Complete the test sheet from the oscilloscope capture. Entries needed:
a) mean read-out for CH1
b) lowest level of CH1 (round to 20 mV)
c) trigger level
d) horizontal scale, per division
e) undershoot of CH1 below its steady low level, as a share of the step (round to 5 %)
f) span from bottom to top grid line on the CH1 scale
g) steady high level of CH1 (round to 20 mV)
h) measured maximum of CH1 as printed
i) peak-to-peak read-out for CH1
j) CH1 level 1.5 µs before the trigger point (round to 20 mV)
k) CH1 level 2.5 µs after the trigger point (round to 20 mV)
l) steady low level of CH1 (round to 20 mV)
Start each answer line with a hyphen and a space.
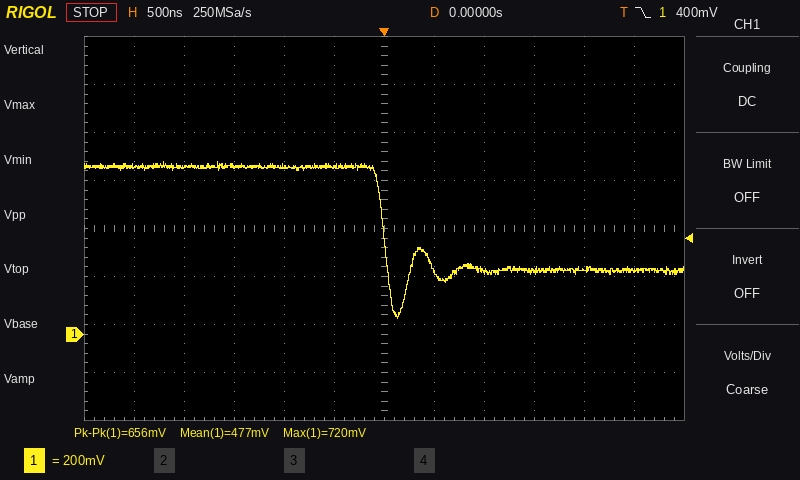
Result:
- 477 mV
- 60 mV
- 400 mV
- 500 ns
- 45 %
- 1.6 V
- 700 mV
- 720 mV
- 656 mV
- 700 mV
- 260 mV
- 260 mV
